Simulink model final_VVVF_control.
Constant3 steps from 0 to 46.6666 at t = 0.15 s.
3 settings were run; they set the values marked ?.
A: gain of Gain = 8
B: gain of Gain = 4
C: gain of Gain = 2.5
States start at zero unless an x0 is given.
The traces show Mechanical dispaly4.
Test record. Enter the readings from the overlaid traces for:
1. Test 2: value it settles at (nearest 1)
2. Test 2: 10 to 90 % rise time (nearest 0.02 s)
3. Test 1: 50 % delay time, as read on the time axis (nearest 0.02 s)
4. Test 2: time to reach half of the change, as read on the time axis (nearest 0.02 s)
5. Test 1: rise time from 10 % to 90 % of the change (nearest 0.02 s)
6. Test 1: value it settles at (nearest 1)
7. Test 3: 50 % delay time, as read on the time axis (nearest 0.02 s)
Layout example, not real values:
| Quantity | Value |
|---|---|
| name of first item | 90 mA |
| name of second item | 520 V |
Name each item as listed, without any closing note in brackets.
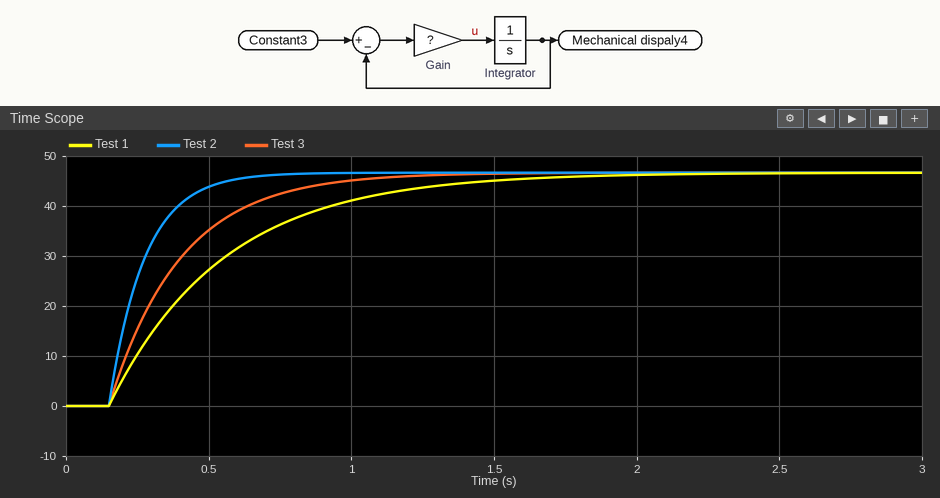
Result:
| Quantity | Value |
|---|---|
| Test 2: value it settles at | 47 |
| Test 2: 10 to 90 % rise time | 0.28 s |
| Test 1: 50 % delay time, as read on the time axis | 0.42 s |
| Test 2: time to reach half of the change, as read on the time axis | 0.24 s |
| Test 1: rise time from 10 % to 90 % of the change | 0.88 s |
| Test 1: value it settles at | 47 |
| Test 3: 50 % delay time, as read on the time axis | 0.32 s |
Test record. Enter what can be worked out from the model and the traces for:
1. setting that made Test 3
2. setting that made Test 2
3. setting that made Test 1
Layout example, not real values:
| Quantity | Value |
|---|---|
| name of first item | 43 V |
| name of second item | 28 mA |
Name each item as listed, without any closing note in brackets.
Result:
| Quantity | Value |
|---|---|
| setting that made Test 3 | B |
| setting that made Test 2 | A |
| setting that made Test 1 | C |
